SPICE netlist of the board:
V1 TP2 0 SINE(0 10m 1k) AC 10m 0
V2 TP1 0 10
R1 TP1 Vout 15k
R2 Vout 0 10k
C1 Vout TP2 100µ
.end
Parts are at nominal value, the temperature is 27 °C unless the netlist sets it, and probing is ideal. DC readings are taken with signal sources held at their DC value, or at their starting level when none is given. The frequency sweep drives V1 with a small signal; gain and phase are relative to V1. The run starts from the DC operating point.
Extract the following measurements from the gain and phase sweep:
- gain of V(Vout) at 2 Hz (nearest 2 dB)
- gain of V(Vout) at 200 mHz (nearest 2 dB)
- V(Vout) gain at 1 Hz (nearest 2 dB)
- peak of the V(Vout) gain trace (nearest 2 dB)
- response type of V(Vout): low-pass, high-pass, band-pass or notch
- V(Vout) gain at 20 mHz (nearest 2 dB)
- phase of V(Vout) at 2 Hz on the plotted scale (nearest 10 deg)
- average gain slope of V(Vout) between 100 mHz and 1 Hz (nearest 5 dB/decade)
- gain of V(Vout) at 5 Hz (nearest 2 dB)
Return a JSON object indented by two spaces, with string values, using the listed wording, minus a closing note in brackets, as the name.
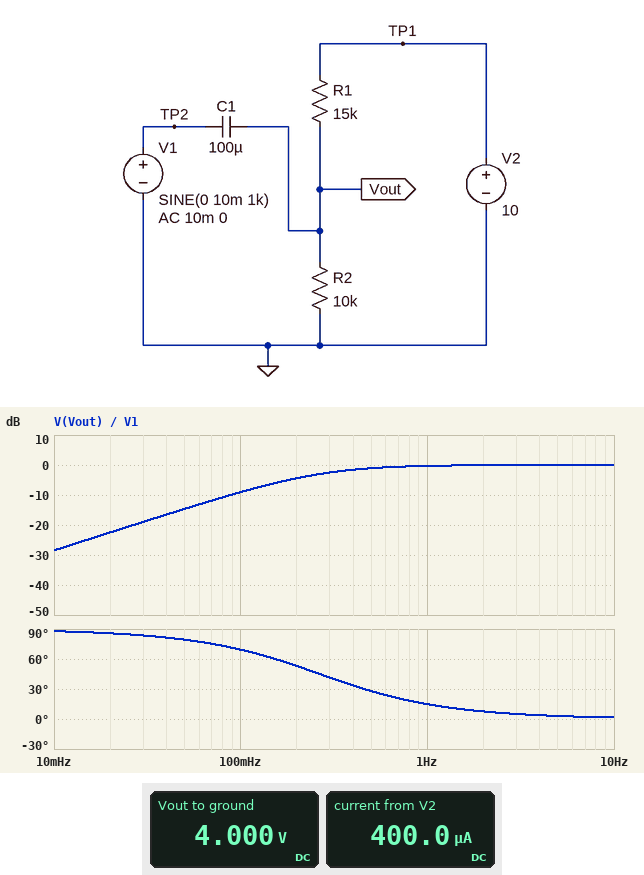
{
  "gain of V(Vout) at 2 Hz": "0 dB",
  "gain of V(Vout) at 200 mHz": "-4 dB",
  "V(Vout) gain at 1 Hz": "0 dB",
  "peak of the V(Vout) gain trace": "0 dB",
  "response type of V(Vout): low-pass, high-pass, band-pass or notch": "high-pass",
  "V(Vout) gain at 20 mHz": "-22 dB",
  "phase of V(Vout) at 2 Hz on the plotted scale": "10 deg",
  "average gain slope of V(Vout) between 100 mHz and 1 Hz": "10 dB/decade",
  "gain of V(Vout) at 5 Hz": "0 dB"
}
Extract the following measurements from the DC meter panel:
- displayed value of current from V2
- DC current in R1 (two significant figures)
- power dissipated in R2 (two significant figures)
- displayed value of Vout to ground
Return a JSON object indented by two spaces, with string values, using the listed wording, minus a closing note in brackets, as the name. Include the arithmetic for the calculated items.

{
  "displayed value of current from V2": "400.0 µA",
  "DC current in R1": "(10 V - 4 V) / 15 kΩ = 400 µA",
  "power dissipated in R2": "(4 V)^2 / 10 kΩ = 1.6 mW",
  "displayed value of Vout to ground": "4.000 V"
}
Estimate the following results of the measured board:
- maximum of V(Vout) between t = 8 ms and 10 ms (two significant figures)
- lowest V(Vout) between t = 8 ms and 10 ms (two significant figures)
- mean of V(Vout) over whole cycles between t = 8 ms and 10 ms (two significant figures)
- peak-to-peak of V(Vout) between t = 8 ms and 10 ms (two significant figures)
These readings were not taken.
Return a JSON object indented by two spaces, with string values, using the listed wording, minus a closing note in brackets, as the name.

{
  "maximum of V(Vout) between t = 8 ms and 10 ms": "4.0 V",
  "lowest V(Vout) between t = 8 ms and 10 ms": "4.0 V",
  "mean of V(Vout) over whole cycles between t = 8 ms and 10 ms": "4.0 V",
  "peak-to-peak of V(Vout) between t = 8 ms and 10 ms": "20 mV"
}
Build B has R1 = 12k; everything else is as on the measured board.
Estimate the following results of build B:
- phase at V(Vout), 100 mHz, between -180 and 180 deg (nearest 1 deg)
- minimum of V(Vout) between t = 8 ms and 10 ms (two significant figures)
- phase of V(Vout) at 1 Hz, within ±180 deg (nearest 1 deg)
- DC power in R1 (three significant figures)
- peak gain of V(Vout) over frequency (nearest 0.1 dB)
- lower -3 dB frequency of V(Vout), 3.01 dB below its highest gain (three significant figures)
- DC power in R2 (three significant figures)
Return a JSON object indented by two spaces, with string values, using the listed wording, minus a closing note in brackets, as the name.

{
  "phase at V(Vout), 100 mHz, between -180 and 180 deg": "71 deg",
  "minimum of V(Vout) between t = 8 ms and 10 ms": "4.5 V",
  "phase of V(Vout) at 1 Hz, within ±180 deg": "16 deg",
  "DC power in R1": "2.48 mW",
  "peak gain of V(Vout) over frequency": "0 dB",
  "lower -3 dB frequency of V(Vout), 3.01 dB below its highest gain": "292 mHz",
  "DC power in R2": "2.07 mW"
}
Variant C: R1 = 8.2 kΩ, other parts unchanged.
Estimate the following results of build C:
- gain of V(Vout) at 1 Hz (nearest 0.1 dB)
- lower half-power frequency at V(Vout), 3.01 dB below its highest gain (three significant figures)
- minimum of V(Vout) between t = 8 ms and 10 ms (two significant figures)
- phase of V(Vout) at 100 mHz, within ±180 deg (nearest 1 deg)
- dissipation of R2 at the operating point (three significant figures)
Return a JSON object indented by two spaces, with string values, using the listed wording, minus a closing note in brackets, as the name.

{
  "gain of V(Vout) at 1 Hz": "-0.5 dB",
  "lower half-power frequency at V(Vout), 3.01 dB below its highest gain": "353 mHz",
  "minimum of V(Vout) between t = 8 ms and 10 ms": "5.5 V",
  "phase of V(Vout) at 100 mHz, within ±180 deg": "74 deg",
  "dissipation of R2 at the operating point": "3.02 mW"
}
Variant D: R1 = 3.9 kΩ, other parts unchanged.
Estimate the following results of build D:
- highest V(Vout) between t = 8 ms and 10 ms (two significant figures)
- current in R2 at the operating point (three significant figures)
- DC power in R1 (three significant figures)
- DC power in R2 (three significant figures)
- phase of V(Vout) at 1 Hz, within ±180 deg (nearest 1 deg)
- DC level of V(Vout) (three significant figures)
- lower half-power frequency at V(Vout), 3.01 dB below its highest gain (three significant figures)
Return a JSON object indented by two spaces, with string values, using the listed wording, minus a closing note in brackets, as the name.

{
  "highest V(Vout) between t = 8 ms and 10 ms": "7.2 V",
  "current in R2 at the operating point": "719 µA",
  "DC power in R1": "2.02 mW",
  "DC power in R2": "5.18 mW",
  "phase of V(Vout) at 1 Hz, within ±180 deg": "30 deg",
  "DC level of V(Vout)": "7.19 V",
  "lower half-power frequency at V(Vout), 3.01 dB below its highest gain": "567 mHz"
}
